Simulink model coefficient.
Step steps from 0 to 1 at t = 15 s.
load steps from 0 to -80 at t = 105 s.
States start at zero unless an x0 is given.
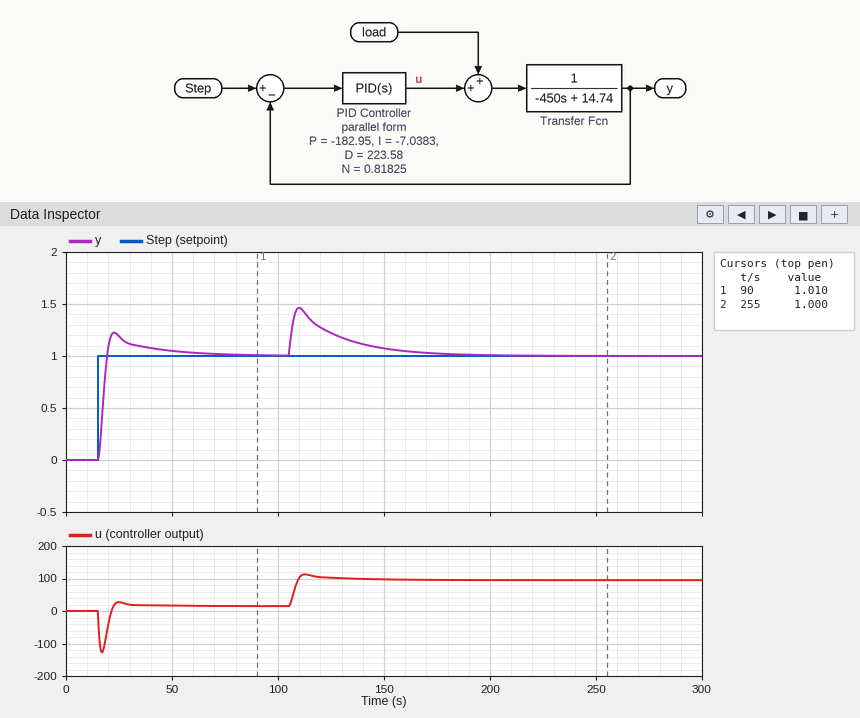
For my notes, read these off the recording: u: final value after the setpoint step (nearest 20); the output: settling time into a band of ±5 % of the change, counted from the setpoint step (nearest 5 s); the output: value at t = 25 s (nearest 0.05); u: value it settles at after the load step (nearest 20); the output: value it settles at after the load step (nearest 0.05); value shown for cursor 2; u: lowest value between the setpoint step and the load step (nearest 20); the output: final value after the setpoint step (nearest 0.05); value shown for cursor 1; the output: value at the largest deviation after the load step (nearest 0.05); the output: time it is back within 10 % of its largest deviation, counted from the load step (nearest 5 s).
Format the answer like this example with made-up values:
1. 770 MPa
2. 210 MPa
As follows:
1. 20
2. 35 s
3. 1.20
4. 100
5. 1.00
6. 1.000
7. -120
8. 1.00
9. 1.010
10. 1.45
11. 55 s
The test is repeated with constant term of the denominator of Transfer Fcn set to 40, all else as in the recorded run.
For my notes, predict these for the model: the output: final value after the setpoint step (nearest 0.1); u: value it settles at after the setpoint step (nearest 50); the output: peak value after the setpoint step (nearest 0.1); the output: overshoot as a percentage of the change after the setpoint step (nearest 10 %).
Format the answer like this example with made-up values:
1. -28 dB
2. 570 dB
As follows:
1. 1.0
2. 50
3. 1.4
4. 40 %
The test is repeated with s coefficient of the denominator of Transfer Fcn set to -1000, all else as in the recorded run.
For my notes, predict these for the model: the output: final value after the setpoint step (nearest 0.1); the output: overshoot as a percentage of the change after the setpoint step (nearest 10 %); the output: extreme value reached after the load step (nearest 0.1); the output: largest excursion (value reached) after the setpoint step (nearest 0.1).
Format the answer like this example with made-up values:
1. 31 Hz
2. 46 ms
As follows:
1. 1.0
2. 20 %
3. 1.4
4. 1.2
